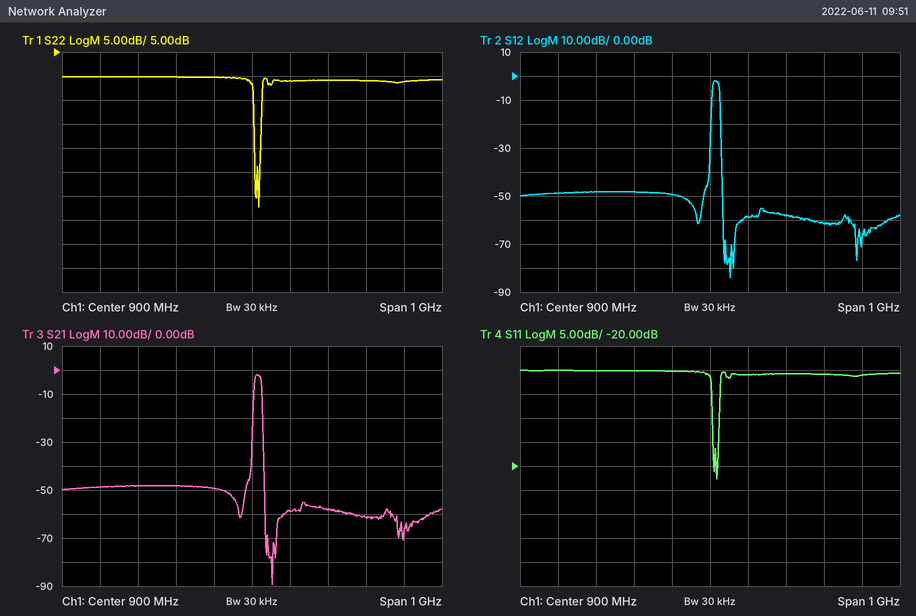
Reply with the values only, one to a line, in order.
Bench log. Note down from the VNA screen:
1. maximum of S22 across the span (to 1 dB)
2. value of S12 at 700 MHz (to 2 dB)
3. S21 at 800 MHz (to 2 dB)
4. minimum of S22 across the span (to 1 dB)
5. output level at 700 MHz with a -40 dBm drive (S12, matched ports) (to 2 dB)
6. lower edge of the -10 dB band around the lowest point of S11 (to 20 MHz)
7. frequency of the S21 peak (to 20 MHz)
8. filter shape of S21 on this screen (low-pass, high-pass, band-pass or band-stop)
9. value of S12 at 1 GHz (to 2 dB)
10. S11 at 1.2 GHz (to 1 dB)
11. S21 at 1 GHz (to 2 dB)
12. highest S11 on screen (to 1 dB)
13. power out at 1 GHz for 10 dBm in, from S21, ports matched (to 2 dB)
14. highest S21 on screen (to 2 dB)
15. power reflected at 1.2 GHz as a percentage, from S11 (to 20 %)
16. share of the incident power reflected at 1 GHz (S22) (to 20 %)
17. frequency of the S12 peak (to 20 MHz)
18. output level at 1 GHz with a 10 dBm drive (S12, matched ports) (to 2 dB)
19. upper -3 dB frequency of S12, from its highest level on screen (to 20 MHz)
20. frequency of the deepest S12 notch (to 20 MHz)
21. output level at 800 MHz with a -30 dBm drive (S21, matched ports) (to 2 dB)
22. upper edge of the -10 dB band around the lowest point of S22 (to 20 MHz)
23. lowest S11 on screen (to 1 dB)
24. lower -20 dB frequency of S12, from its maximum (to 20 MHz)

0 dB
-48 dB
-50 dB
-27 dB
-88 dBm
900 MHz
920 MHz
band-pass
-58 dB
-1 dB
-58 dB
0 dB
-48 dBm
-2 dB
80 %
80 %
920 MHz
-48 dBm
920 MHz
960 MHz
-80 dBm
920 MHz
-23 dB
900 MHz
